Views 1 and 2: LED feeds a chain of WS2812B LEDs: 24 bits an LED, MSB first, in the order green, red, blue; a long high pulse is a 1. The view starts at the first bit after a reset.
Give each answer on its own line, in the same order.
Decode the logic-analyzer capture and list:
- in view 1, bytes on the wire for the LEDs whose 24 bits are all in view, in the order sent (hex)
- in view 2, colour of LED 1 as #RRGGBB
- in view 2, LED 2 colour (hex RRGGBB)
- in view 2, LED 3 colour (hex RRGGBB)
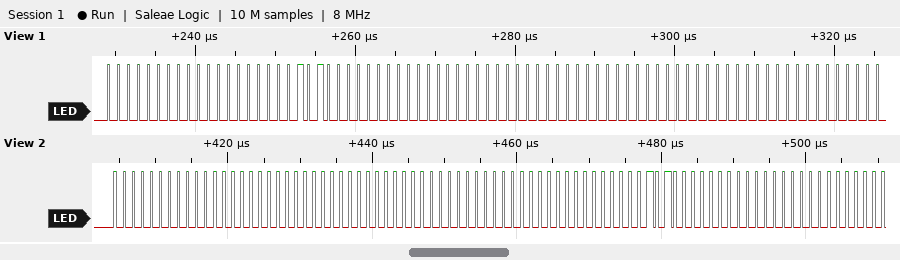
00 00 14 00 00 00 00 00 00
#000000
#000000
#140000
